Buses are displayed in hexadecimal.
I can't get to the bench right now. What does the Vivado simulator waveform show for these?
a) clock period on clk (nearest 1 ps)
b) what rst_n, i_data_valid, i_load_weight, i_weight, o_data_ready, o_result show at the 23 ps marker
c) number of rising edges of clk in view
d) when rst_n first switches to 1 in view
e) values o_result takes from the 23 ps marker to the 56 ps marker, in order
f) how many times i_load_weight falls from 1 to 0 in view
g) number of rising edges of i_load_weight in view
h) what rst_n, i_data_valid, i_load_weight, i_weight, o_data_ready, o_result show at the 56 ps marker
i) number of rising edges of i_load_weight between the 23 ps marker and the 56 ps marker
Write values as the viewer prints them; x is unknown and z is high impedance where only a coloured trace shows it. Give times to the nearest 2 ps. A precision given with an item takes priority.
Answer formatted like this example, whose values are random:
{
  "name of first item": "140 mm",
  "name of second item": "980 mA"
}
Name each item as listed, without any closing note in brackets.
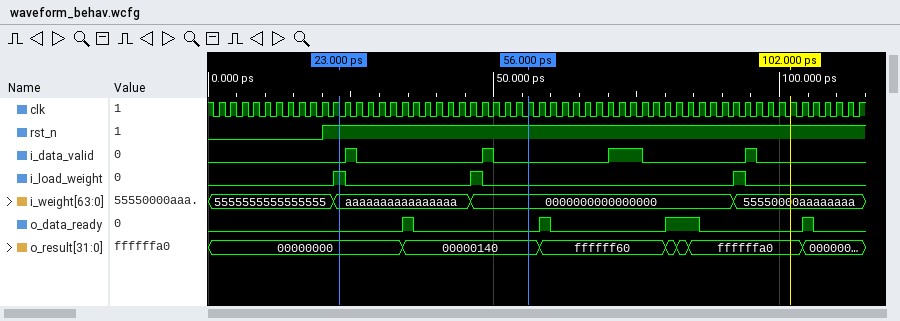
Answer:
{
  "clock period on clk": "2 ps",
  "what rst_n, i_data_valid, i_load_weight, i_weight, o_data_ready, o_result show at the 23 ps marker": "rst_n=1, i_data_valid=0, i_load_weight=1, i_weight=aaaaaaaaaaaaaaaa, o_data_ready=0, o_result=00000000",
  "number of rising edges of clk in view": "57",
  "when rst_n first switches to 1 in view": "20 ps",
  "values o_result takes from the 23 ps marker to the 56 ps marker, in order": "00000000, 00000140",
  "how many times i_load_weight falls from 1 to 0 in view": "3",
  "number of rising edges of i_load_weight in view": "3",
  "what rst_n, i_data_valid, i_load_weight, i_weight, o_data_ready, o_result show at the 56 ps marker": "rst_n=1, i_data_valid=0, i_load_weight=0, i_weight=0000000000000000, o_data_ready=0, o_result=00000140",
  "number of rising edges of i_load_weight between the 23 ps marker and the 56 ps marker": "1"
}
